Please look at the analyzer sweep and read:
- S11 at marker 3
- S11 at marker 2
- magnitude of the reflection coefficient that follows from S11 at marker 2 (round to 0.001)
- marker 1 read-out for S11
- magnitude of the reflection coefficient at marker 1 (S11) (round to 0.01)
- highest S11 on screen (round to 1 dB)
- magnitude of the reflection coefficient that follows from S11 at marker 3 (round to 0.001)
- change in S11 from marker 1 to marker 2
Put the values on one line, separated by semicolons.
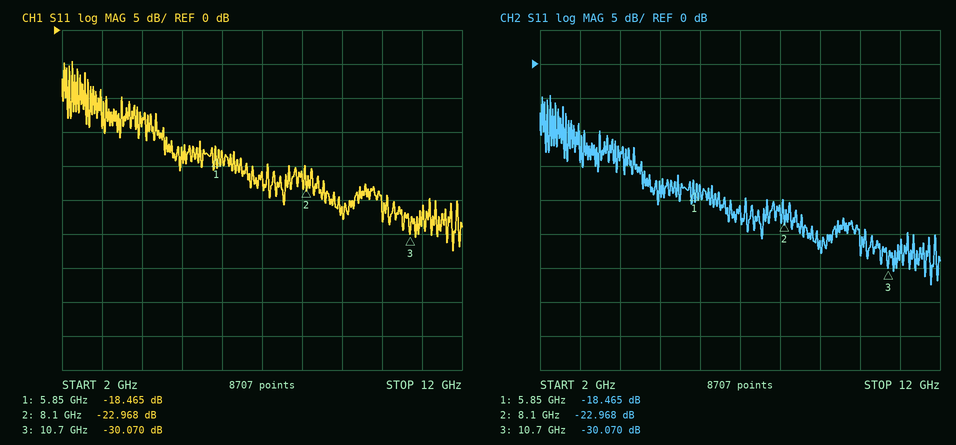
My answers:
-30.070 dB; -22.968 dB; 0.071; -18.465 dB; 0.12; -5 dB; 0.031; -4.503 dB
